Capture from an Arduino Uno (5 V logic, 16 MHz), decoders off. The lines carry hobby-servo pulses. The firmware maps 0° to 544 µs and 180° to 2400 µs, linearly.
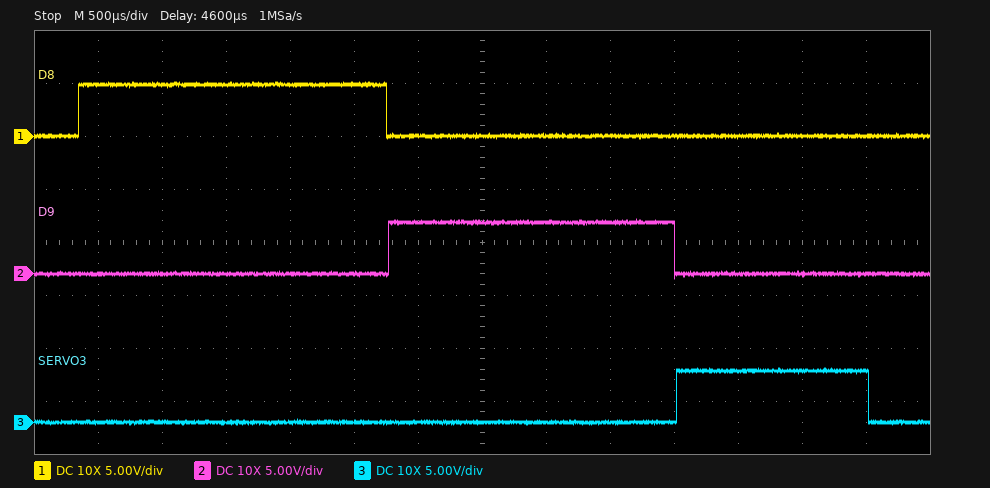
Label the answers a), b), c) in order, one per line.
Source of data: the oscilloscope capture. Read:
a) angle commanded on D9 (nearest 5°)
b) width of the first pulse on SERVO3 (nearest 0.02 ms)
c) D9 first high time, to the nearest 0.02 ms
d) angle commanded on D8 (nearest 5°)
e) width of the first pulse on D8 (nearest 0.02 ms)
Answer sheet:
a) 165°
b) 1.50 ms
c) 2.24 ms
d) 180°
e) 2.40 ms
